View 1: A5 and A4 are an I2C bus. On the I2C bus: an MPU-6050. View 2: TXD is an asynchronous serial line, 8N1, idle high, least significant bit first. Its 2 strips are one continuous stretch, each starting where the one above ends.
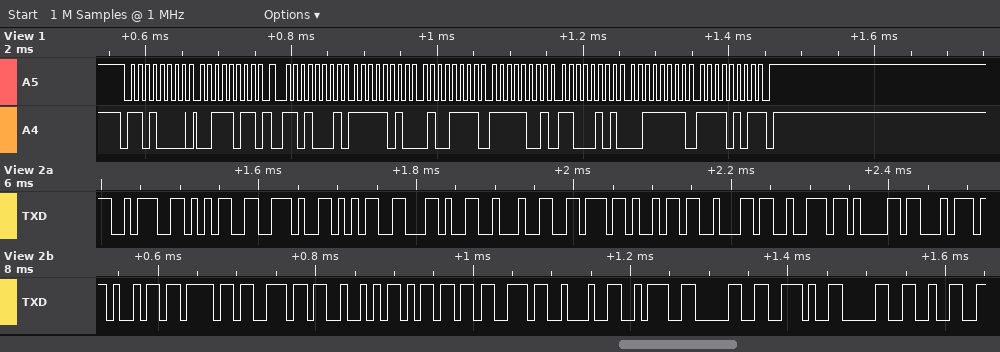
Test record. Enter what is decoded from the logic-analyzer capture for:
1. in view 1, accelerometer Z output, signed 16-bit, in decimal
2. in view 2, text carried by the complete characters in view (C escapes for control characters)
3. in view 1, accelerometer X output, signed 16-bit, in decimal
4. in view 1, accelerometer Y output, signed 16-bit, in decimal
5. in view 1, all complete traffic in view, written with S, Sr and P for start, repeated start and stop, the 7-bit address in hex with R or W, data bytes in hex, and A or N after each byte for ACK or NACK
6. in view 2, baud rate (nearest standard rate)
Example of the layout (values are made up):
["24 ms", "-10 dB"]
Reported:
["16373", "\":5.5,\\\"vibrationRms\\\":0.02\"", "-1457", "-1595", "S 68W A 3B A Sr 68R A FA A 4F A F9 A C5 A 3F A F5 N P", "115200 baud"]
